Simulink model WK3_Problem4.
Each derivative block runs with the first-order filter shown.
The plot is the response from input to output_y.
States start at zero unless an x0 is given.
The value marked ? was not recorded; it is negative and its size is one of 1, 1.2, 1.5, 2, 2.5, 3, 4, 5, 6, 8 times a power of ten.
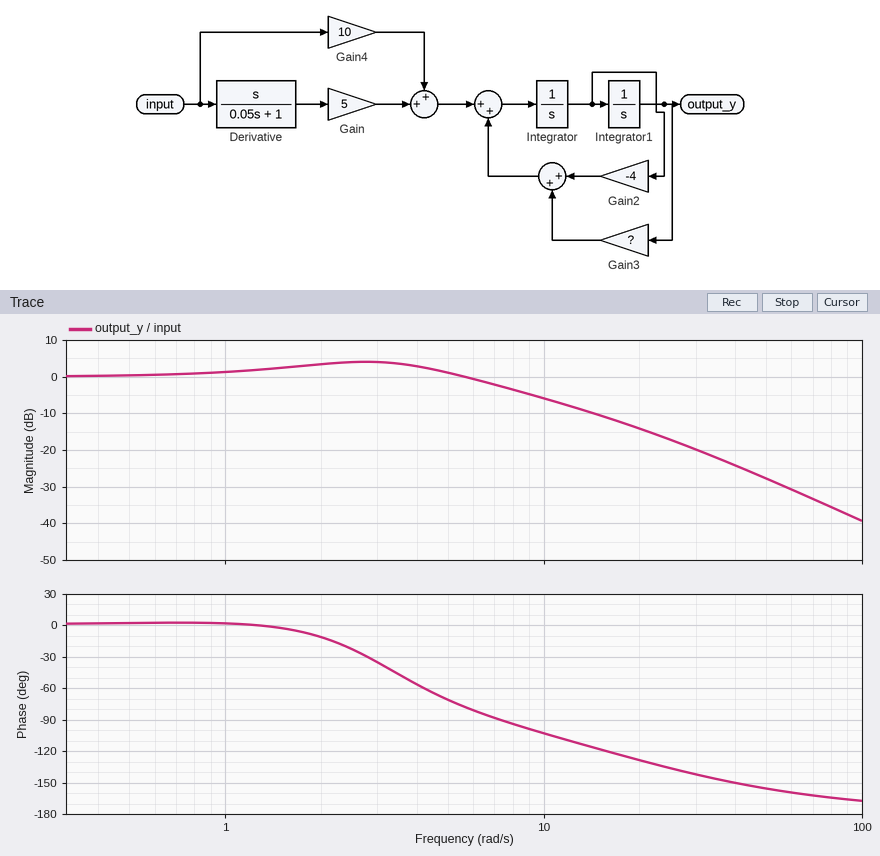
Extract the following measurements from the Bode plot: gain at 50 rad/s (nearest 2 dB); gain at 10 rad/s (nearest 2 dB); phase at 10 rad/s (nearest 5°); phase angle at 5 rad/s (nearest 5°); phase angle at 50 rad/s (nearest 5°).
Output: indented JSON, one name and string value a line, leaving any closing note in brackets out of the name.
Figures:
{
  "gain at 50 rad/s": "-28 dB",
  "gain at 10 rad/s": "-6 dB",
  "phase at 10 rad/s": "-105°",
  "phase angle at 5 rad/s": "-70°",
  "phase angle at 50 rad/s": "-155°"
}
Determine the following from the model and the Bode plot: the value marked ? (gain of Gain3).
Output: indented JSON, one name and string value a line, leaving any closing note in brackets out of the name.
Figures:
{
  "the value marked ?": "-10"
}
